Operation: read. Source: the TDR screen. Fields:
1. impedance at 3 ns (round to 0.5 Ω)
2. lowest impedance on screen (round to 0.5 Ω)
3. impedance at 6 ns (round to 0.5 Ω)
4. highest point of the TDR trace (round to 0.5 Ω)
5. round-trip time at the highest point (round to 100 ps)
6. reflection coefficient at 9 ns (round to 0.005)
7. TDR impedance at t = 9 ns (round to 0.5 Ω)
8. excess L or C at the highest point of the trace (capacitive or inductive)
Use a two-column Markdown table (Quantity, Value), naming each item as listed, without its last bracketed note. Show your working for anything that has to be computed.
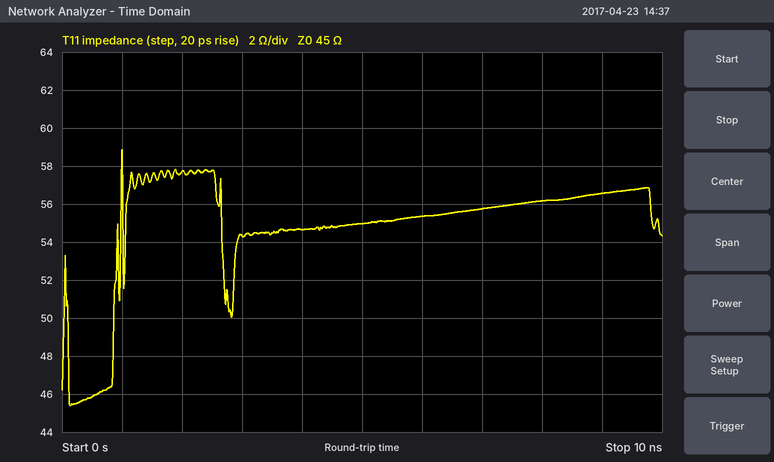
| Quantity | Value |
|---|---|
| impedance at 3 ns | 54.5 Ω |
| lowest impedance on screen | 45.5 Ω |
| impedance at 6 ns | 55.5 Ω |
| highest point of the TDR trace | 59.0 Ω |
| round-trip time at the highest point | 1.0 ns |
| reflection coefficient at 9 ns | (56.5 − 45)/(56.5 + 45) ≈ +0.113, so +0.115 to the nearest 0.005 |
| TDR impedance at t = 9 ns | 56.5 Ω |
| excess L or C at the highest point of the trace | inductive |
